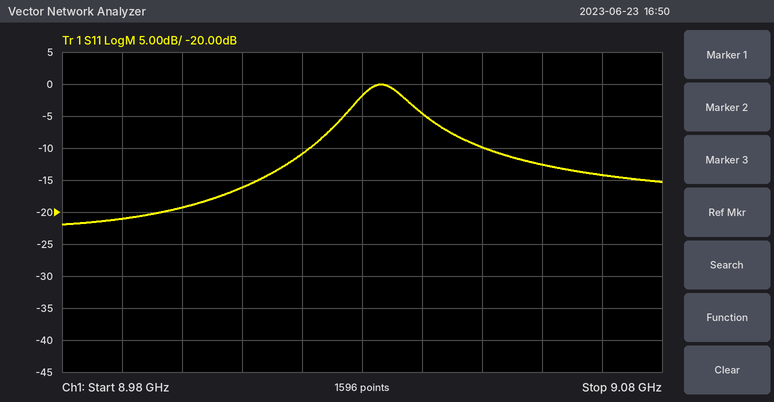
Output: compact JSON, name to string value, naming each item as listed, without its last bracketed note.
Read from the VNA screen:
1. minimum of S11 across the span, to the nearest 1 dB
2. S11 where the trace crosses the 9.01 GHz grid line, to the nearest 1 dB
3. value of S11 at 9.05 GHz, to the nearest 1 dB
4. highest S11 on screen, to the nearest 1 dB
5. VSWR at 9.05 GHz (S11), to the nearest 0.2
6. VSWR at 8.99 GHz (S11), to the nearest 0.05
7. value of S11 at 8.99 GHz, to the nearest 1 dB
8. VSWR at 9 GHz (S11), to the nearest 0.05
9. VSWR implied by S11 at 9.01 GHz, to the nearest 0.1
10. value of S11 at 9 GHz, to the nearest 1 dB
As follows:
{"minimum of S11 across the span, to the nearest 1 dB": "-22 dB", "S11 where the trace crosses the 9.01 GHz grid line, to the nearest 1 dB": "-16 dB", "value of S11 at 9.05 GHz, to the nearest 1 dB": "-10 dB", "highest S11 on screen, to the nearest 1 dB": "0 dB", "VSWR at 9.05 GHz (S11), to the nearest 0.2": "2.0", "VSWR at 8.99 GHz (S11), to the nearest 0.05": "1.20", "value of S11 at 8.99 GHz, to the nearest 1 dB": "-21 dB", "VSWR at 9 GHz (S11), to the nearest 0.05": "1.25", "VSWR implied by S11 at 9.01 GHz, to the nearest 0.1": "1.4", "value of S11 at 9 GHz, to the nearest 1 dB": "-19 dB"}
